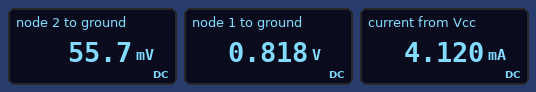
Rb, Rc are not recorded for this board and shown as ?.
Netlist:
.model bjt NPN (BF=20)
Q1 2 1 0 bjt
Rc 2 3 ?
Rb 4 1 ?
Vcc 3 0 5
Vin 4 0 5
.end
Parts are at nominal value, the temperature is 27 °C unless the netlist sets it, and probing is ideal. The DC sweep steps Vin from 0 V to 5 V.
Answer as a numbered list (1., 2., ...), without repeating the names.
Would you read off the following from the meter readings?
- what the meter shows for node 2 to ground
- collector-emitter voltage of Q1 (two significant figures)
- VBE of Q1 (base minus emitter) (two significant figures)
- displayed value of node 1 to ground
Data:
1. 55.7 mV
2. 56 mV
3. 820 mV
4. 0.818 V
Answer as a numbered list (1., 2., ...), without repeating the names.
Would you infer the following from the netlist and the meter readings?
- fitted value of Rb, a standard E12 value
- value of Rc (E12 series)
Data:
1. 4.7 kΩ
2. 1.2 kΩ
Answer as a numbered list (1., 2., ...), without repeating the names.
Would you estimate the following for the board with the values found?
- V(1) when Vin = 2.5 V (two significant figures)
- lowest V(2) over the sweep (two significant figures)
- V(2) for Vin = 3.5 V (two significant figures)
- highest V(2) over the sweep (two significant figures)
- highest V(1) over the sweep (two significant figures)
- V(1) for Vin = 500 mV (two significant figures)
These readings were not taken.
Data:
1. 810 mV
2. 56 mV
3. 69 mV
4. 5.0 V
5. 820 mV
6. 500 mV
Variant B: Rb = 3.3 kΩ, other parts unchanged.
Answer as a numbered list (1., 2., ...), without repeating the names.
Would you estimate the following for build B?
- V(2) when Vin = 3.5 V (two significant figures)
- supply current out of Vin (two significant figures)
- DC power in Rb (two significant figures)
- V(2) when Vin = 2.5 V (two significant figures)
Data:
1. 58 mV
2. 1.3 mA
3. 5.3 mW
4. 73 mV
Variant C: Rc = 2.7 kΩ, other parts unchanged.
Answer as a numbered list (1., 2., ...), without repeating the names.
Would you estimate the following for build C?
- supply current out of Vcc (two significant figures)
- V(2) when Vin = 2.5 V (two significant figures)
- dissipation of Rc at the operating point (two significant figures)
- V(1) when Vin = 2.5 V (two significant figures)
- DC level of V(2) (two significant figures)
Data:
1. 1.8 mA
2. 58 mV
3. 9.1 mW
4. 800 mV
5. 39 mV
